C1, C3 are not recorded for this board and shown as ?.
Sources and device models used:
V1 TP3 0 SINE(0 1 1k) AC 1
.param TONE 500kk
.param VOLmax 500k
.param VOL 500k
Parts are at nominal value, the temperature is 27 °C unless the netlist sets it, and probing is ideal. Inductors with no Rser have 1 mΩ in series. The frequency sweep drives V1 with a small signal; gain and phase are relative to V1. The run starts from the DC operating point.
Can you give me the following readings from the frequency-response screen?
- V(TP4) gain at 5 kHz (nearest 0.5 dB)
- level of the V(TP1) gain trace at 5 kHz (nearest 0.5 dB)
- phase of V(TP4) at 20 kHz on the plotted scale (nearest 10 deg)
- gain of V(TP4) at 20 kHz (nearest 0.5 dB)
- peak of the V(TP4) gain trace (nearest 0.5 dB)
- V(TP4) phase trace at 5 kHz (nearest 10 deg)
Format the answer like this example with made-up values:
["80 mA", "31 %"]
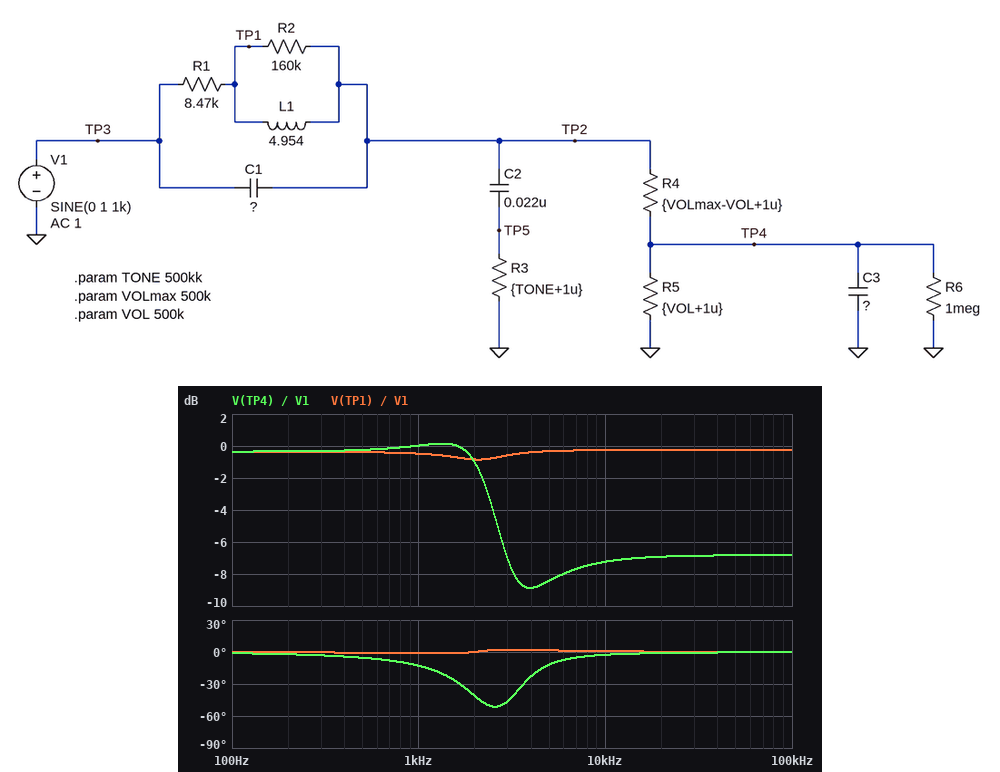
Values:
["-8.5 dB", "-0.5 dB", "0 deg", "-7.0 dB", "0 dB", "-10 deg"]
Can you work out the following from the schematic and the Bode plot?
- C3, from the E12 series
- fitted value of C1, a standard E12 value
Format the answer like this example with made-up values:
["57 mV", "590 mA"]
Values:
["560 pF", "470 pF"]
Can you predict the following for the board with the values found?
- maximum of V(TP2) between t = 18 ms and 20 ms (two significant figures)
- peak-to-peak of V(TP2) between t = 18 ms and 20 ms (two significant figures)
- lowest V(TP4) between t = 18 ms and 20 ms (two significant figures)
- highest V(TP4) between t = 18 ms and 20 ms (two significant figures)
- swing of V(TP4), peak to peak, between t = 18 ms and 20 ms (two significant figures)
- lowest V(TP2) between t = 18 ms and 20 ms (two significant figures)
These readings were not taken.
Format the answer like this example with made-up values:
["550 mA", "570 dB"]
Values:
["1.0 V", "2.0 V", "-1.0 V", "1.0 V", "2.0 V", "-1.0 V"]
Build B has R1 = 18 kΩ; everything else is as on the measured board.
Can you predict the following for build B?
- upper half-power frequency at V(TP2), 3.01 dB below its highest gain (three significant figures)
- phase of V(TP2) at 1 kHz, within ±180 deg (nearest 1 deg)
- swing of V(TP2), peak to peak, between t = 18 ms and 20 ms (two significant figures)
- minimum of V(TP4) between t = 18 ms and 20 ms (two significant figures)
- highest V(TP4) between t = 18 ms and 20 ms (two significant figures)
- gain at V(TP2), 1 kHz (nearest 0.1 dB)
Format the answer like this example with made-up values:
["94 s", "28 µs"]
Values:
["2.26 kHz", "-14 deg", "1.9 V", "-940 mV", "940 mV", "-0.5 dB"]
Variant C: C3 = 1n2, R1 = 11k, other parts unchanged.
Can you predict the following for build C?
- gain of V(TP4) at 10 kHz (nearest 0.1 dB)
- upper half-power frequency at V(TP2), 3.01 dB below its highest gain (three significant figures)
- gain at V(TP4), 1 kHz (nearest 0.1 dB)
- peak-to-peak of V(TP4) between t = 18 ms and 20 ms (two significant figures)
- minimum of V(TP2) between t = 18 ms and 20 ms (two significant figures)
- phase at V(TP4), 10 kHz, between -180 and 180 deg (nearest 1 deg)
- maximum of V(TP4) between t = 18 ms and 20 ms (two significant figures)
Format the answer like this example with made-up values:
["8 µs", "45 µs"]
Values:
["-11.5 dB", "1.93 kHz", "0.8 dB", "2.2 V", "-1.1 V", "-6 deg", "1.1 V"]
